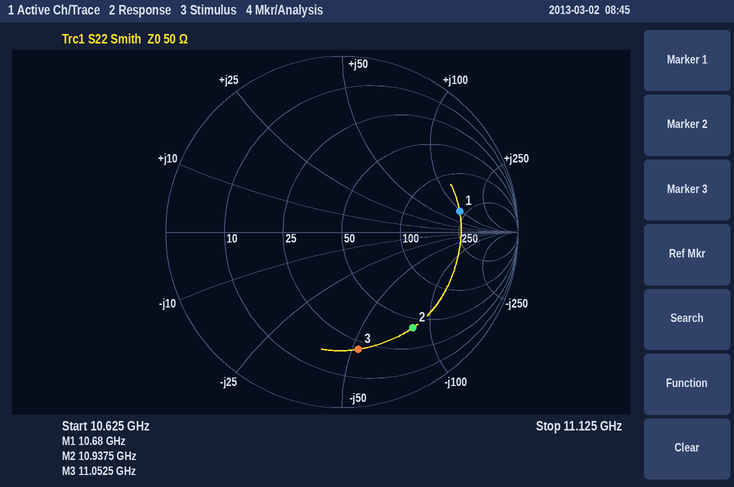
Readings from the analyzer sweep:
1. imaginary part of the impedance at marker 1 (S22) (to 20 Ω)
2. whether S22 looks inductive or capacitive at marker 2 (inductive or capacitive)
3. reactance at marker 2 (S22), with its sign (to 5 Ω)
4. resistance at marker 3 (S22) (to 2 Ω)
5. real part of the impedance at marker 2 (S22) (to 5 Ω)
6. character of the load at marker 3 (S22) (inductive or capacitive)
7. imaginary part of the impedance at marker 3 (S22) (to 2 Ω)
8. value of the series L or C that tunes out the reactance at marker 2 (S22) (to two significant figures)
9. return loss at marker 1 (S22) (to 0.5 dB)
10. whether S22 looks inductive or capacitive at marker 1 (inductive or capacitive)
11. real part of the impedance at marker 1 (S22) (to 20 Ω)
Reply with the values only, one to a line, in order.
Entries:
+100 Ω
capacitive
-85 Ω
22 Ω
40 Ω
capacitive
-52 Ω
1.2 nH
3.5 dB
inductive
220 Ω
